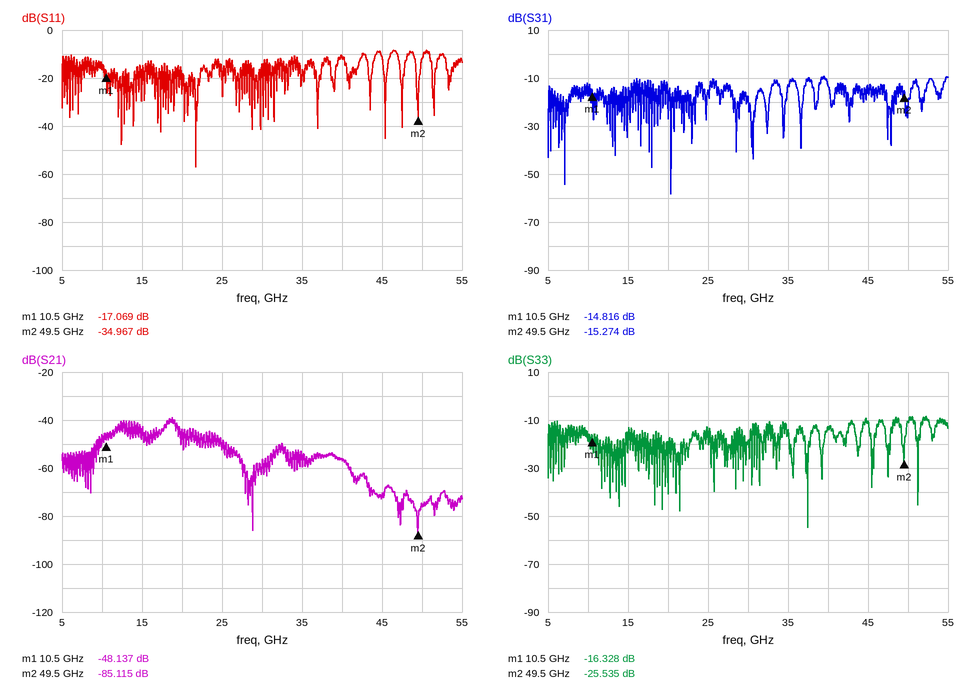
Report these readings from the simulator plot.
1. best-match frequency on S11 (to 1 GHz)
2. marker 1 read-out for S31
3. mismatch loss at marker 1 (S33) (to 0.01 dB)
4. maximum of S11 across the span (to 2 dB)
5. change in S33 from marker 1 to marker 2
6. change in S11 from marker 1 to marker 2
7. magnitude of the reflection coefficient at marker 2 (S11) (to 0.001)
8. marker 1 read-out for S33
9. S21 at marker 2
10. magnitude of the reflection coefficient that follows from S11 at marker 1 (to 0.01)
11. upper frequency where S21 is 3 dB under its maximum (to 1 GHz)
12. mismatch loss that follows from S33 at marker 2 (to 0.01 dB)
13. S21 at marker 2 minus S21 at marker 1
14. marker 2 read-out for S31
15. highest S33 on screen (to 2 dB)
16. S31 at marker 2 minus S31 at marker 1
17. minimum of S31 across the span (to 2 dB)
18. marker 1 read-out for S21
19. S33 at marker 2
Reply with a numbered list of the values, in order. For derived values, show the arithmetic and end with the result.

1. 22 GHz
2. -14.816 dB
3. −10 log10(1 − 10^(-16.328/10)) ≈ 0.10 dB
4. -8 dB
5. -25.535 − (-16.328) = -9.207 dB
6. -34.967 − (-17.069) = -17.898 dB
7. 10^(-34.967/20) ≈ 0.018
8. -16.328 dB
9. -85.115 dB
10. 10^(-17.069/20) ≈ 0.14
11. 19 GHz
12. −10 log10(1 − 10^(-25.535/10)) ≈ 0.01 dB
13. -85.115 − (-48.137) = -36.978 dB
14. -15.274 dB
15. -8 dB
16. -15.274 − (-14.816) = -0.458 dB
17. -58 dB
18. -48.137 dB
19. -25.535 dB
